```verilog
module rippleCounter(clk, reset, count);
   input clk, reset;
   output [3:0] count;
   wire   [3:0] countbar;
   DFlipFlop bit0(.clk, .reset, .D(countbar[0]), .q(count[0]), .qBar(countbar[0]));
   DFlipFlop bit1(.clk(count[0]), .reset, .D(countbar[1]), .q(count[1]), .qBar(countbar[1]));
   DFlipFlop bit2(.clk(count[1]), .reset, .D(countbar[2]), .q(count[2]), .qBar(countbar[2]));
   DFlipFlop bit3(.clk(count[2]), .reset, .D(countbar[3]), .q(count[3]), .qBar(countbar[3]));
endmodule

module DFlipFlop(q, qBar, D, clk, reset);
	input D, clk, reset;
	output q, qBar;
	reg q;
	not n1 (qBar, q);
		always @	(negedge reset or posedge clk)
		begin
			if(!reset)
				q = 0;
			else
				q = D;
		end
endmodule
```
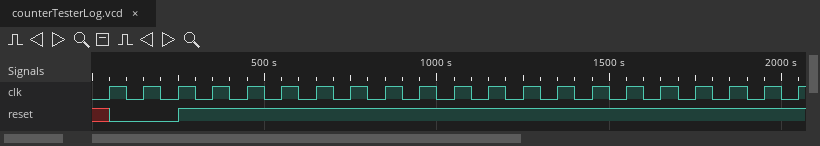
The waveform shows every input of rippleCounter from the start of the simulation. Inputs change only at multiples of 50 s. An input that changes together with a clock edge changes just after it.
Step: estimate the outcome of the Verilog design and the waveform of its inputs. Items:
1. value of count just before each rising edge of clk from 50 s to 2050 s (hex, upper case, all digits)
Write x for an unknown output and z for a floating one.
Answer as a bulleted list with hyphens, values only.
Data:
- x, 0, 0, 0, F, E, D, C, B, A, 9, 8, 7, 6, 5, 4, 3, 2, 1, 0, F
